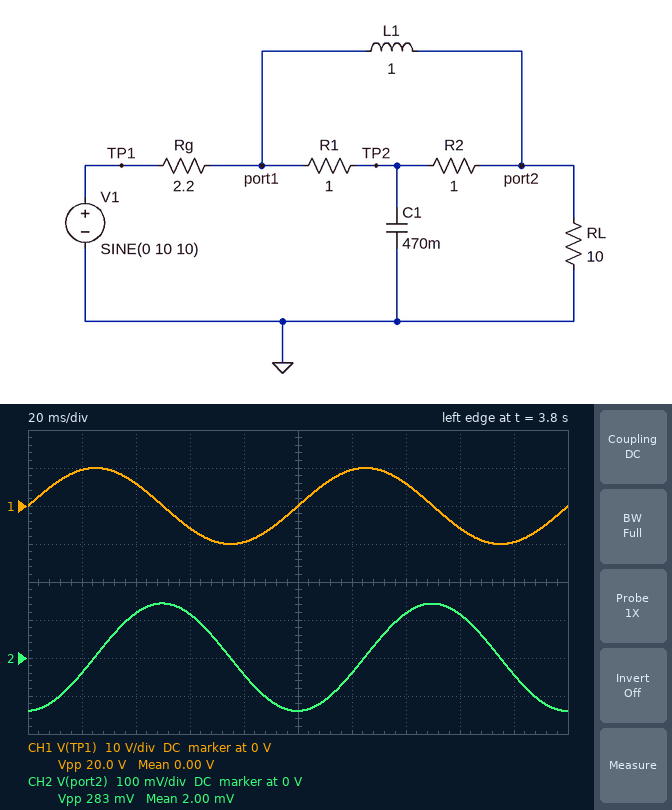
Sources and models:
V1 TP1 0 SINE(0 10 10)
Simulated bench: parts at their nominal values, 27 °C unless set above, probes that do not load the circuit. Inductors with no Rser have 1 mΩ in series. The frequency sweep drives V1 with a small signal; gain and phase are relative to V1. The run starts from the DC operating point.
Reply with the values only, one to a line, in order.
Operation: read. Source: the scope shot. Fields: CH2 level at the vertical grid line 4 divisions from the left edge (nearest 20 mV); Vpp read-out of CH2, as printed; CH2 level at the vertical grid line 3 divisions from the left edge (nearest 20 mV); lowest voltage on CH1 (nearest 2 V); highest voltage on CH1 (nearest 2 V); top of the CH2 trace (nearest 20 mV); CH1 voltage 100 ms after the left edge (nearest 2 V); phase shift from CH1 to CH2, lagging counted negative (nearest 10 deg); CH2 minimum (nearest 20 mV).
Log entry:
-40 mV
283 mV
120 mV
-10 V
10 V
140 mV
0 V
-90 deg
-140 mV
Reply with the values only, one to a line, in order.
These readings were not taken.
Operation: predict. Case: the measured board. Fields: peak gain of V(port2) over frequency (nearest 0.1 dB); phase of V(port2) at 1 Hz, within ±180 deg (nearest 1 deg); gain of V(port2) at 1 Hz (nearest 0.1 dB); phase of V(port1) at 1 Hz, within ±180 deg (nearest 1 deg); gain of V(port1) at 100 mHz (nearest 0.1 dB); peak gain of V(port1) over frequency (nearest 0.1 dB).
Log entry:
-1.7 dB
-80 deg
-17.1 dB
-8 deg
-3.5 dB
-1.7 dB
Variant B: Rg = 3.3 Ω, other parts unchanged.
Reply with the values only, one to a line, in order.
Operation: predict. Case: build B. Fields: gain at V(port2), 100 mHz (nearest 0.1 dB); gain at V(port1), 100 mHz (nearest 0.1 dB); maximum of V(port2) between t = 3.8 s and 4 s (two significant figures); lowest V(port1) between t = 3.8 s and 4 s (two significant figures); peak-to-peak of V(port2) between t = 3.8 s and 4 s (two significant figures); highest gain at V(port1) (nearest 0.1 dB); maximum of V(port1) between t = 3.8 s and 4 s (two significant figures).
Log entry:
-4.6 dB
-5.1 dB
110 mV
-2.3 V
210 mV
-2.5 dB
2.3 V
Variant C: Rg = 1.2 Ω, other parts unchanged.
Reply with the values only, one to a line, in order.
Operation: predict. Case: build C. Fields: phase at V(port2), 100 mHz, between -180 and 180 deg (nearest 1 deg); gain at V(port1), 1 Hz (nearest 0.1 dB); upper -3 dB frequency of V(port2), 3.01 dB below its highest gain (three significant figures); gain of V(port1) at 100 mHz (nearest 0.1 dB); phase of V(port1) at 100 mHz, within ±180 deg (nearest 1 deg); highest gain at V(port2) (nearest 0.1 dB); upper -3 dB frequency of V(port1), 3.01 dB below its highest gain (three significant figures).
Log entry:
-21 deg
-6.8 dB
262 mHz
-1.9 dB
-16 deg
-1.0 dB
206 mHz
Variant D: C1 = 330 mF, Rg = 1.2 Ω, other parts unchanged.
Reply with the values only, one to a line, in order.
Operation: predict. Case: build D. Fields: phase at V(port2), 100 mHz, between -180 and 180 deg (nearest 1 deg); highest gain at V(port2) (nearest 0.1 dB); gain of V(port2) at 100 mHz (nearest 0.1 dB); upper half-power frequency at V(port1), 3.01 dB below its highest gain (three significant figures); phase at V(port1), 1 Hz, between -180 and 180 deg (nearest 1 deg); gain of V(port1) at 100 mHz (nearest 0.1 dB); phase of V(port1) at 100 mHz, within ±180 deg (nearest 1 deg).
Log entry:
-16 deg
-1.0 dB
-1.2 dB
298 mHz
-10 deg
-1.5 dB
-12 deg
